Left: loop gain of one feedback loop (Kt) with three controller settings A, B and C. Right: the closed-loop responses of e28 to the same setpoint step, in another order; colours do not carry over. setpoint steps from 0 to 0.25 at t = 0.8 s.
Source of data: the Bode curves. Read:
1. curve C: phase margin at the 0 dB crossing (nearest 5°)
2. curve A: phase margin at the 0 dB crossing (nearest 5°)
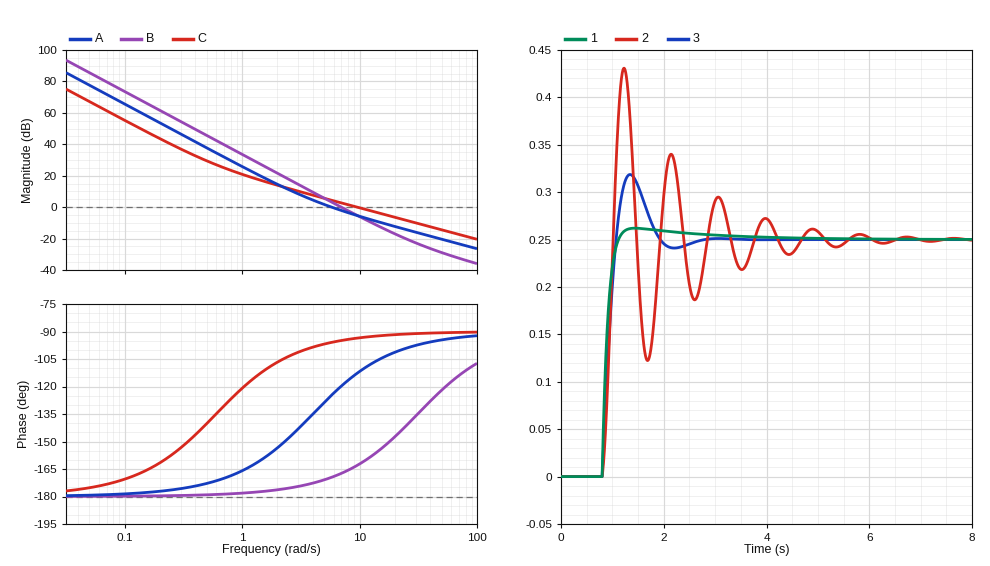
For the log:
85°
55°
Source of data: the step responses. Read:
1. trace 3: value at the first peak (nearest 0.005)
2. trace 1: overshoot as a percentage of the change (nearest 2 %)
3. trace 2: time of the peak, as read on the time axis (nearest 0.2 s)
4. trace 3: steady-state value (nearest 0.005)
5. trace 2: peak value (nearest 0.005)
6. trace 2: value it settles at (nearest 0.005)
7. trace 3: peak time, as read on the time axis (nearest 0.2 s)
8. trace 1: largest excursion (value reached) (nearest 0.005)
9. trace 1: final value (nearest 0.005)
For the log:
0.320
4 %
1.2 s
0.250
0.430
0.250
1.4 s
0.260
0.250
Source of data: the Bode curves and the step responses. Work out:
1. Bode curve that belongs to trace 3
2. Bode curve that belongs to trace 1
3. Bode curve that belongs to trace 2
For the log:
A
C
B
